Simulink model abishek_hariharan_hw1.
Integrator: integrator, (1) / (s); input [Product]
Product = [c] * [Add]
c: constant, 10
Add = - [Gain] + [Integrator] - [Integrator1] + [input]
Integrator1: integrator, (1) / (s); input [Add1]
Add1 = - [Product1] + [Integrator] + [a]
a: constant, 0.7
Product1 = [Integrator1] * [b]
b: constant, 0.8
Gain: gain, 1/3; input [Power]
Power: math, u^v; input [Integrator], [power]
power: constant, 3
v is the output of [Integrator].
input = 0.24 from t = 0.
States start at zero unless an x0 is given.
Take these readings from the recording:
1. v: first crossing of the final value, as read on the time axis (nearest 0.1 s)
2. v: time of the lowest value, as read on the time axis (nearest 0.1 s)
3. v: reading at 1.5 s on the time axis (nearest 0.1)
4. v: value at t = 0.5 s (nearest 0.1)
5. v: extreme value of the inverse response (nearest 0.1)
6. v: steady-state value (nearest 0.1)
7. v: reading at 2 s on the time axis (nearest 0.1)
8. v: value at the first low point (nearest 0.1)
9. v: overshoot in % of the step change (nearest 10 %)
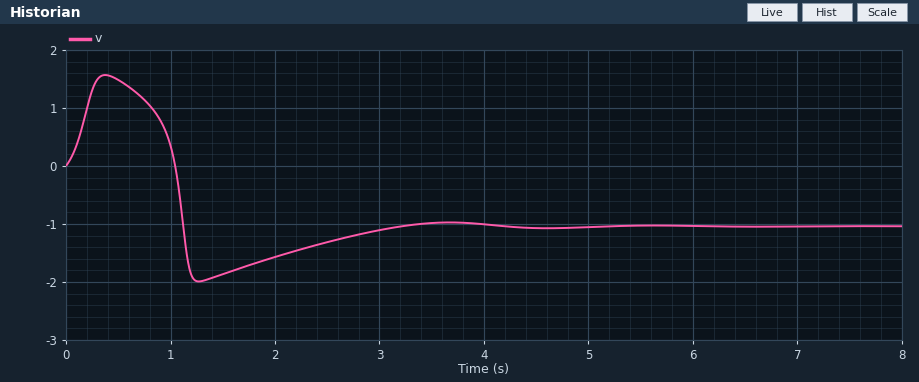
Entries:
1.1 s
1.3 s
-1.9
1.5
1.6
-1.0
-1.6
-2.0
90 %
